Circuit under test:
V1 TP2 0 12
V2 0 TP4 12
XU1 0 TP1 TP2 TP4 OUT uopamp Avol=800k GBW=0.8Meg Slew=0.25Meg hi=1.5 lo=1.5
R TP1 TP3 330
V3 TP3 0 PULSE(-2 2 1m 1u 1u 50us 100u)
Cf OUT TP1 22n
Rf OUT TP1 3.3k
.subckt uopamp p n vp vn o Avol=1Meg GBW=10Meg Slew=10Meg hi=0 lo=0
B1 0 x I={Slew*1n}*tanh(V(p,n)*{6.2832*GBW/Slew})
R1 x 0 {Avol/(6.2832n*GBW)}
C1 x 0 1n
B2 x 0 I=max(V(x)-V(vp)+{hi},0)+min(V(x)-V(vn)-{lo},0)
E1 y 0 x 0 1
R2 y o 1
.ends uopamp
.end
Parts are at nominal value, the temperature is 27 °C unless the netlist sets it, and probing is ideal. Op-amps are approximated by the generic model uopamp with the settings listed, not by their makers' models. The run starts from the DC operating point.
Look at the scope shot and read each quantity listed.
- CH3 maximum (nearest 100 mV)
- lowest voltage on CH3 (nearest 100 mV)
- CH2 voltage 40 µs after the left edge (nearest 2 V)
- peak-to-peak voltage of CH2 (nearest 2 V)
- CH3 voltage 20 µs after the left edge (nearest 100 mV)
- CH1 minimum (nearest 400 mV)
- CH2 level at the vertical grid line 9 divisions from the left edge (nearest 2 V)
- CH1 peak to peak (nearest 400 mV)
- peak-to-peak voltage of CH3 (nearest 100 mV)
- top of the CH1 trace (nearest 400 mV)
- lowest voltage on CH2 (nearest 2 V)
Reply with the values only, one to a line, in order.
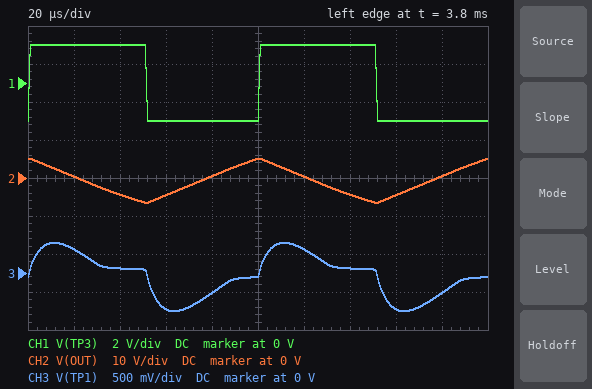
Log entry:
400 mV
-500 mV
-4 V
12 V
300 mV
-2.0 V
0 V
4.0 V
900 mV
2.0 V
-6 V
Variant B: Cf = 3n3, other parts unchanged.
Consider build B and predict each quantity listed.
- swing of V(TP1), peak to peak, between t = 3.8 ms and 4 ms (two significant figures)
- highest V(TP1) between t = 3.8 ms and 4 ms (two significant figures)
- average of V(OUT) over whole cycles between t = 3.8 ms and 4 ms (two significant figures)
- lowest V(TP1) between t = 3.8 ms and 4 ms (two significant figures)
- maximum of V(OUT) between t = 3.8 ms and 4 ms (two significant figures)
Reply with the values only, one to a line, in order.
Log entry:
4.1 V
1.6 V
-4.4 V
-2.4 V
1.8 V
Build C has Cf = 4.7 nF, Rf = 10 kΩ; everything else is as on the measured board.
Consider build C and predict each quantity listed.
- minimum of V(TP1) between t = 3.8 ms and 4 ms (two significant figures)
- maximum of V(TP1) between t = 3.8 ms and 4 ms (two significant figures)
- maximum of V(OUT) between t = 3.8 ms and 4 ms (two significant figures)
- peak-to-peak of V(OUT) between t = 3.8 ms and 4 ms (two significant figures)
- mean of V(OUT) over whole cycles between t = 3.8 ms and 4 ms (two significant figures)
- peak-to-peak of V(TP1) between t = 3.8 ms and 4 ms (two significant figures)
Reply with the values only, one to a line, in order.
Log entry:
-1.8 V
1.6 V
1.7 V
12 V
-4.5 V
3.4 V
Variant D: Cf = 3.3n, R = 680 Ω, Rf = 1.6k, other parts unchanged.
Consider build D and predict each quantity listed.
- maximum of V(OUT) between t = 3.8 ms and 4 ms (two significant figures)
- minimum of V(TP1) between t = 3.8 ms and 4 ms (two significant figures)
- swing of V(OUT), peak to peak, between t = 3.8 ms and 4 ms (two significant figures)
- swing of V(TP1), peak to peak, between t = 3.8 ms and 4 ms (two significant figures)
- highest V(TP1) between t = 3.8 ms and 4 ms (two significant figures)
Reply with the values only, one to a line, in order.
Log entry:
4.6 V
-2.0 V
9.3 V
4.0 V
2.0 V
